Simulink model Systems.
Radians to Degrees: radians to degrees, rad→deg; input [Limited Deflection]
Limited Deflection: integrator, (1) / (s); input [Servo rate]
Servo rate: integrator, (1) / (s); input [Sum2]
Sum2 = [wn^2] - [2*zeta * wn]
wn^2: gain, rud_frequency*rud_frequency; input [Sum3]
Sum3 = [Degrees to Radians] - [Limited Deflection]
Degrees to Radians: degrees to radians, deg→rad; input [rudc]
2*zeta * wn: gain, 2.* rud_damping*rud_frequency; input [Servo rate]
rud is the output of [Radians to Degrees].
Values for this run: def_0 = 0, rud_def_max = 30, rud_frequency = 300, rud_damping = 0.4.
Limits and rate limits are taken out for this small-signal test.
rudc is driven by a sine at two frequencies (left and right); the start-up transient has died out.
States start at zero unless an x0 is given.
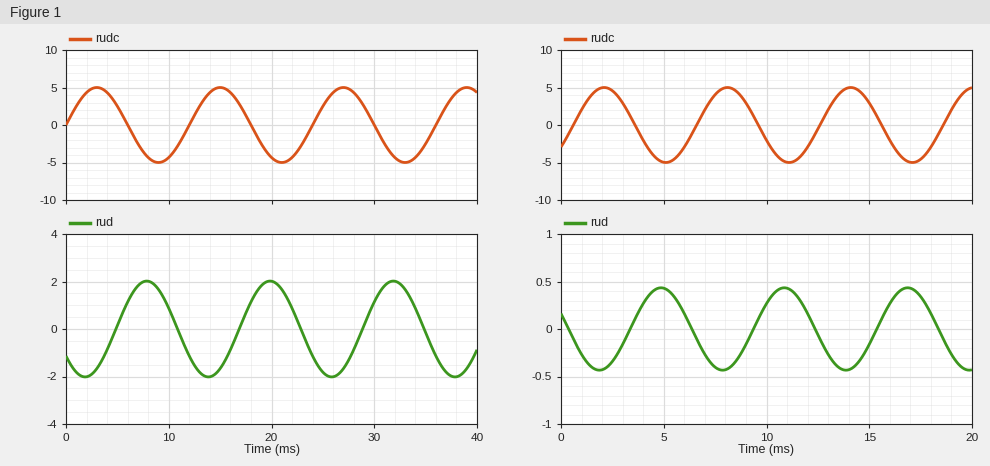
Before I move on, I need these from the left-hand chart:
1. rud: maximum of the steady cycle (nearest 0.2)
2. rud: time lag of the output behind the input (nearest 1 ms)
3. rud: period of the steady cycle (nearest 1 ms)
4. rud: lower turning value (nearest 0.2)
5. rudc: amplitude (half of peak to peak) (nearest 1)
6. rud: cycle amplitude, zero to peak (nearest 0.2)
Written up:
2.0
5 ms
12 ms
-2.0
5
2.0
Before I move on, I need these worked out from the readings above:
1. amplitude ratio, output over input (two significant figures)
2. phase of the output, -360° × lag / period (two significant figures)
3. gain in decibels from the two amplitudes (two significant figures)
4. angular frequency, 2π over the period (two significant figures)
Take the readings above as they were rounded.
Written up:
0.40
-150°
-8.0 dB
0.52 rad/ms
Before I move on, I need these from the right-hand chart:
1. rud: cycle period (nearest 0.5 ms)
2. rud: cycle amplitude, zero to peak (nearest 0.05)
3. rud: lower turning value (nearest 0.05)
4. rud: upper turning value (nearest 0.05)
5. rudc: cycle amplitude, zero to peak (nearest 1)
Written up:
6.0 ms
0.45
-0.45
0.45
5
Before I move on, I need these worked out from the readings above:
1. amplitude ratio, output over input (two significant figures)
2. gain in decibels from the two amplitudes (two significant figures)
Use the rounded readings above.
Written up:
0.090
-21 dB
